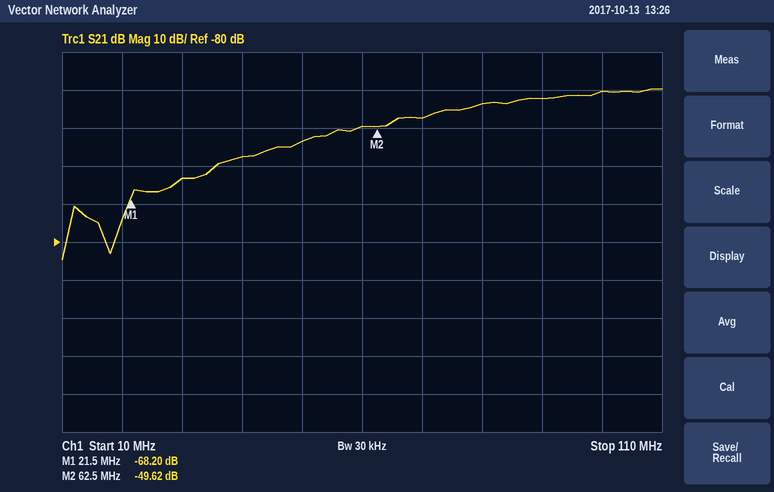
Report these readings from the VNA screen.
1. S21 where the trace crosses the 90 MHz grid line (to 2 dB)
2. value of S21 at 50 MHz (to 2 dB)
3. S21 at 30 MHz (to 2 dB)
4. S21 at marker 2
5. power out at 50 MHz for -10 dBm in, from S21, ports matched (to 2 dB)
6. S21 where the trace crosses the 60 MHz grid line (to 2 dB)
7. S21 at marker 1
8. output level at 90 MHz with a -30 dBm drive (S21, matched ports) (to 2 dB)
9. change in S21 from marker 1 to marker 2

-42 dB
-54 dB
-64 dB
-49.62 dB
-64 dBm
-50 dB
-68.20 dB
-72 dBm
18.58 dB
